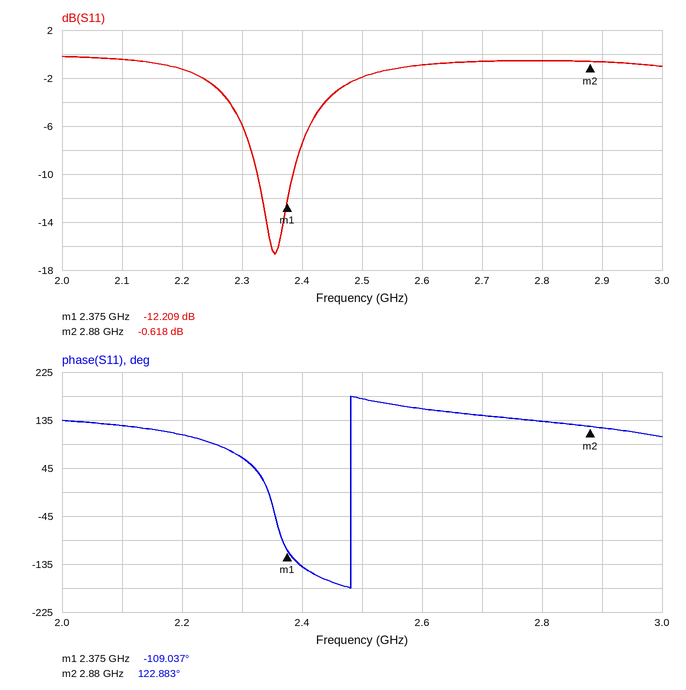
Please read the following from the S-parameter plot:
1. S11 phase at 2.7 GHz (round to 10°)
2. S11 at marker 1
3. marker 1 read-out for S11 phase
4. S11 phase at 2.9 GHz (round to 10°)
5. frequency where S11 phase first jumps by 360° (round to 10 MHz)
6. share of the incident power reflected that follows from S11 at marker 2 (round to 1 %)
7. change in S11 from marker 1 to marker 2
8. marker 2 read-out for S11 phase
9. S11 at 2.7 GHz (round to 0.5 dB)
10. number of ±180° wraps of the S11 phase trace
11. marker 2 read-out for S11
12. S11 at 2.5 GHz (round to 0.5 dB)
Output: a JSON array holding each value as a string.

["140°", "-12.209 dB", "-109.037°", "120°", "2.48 GHz", "87 %", "11.591 dB", "122.883°", "-0.5 dB", "1", "-0.618 dB", "-2.0 dB"]
